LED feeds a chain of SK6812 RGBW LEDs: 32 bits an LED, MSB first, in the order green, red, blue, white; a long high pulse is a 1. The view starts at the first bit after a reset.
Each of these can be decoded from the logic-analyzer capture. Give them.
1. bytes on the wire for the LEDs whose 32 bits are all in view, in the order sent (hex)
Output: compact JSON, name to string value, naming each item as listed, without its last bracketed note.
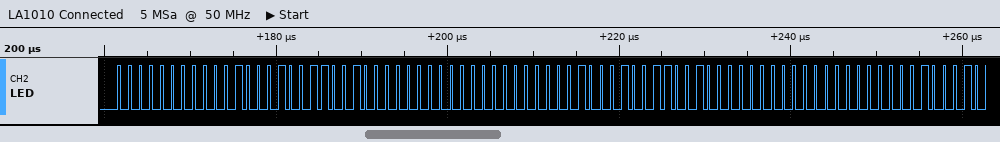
{"bytes on the wire for the LEDs whose 32 bits are all in view, in the order sent": "00 11 32 00 00 11 32 00"}
